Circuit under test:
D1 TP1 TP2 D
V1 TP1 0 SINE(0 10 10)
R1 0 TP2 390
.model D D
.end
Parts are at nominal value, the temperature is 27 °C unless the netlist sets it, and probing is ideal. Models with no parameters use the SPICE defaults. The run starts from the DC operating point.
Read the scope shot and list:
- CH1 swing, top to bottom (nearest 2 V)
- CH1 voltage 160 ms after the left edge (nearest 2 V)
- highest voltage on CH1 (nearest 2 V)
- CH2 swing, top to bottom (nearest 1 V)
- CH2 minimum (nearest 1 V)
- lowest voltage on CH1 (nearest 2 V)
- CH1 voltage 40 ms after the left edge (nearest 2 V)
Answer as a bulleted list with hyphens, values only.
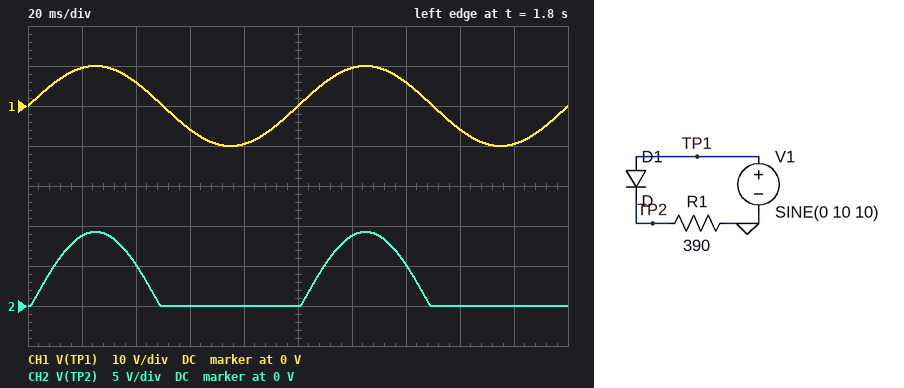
- 20 V
- -6 V
- 10 V
- 9 V
- 0 V
- -10 V
- 6 V
